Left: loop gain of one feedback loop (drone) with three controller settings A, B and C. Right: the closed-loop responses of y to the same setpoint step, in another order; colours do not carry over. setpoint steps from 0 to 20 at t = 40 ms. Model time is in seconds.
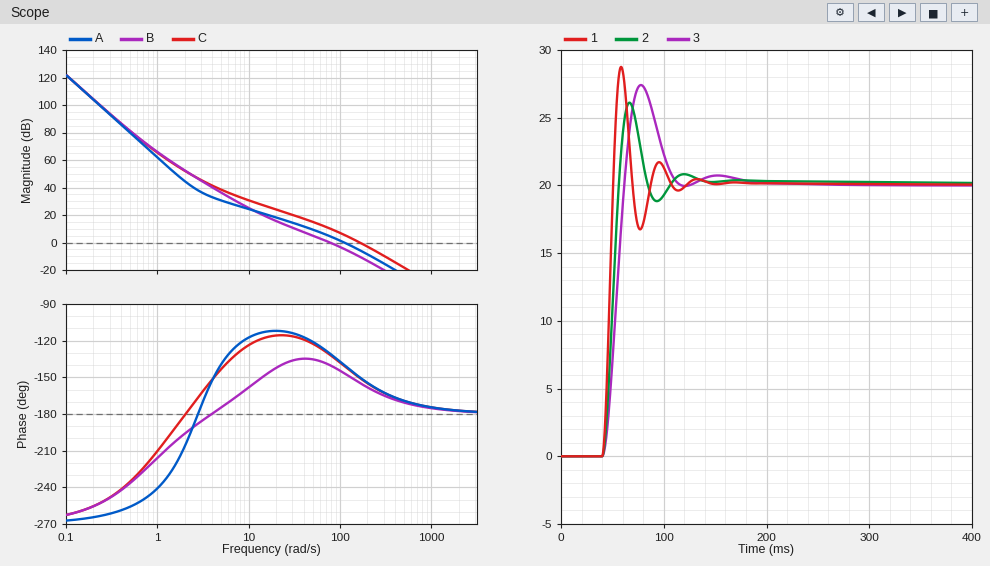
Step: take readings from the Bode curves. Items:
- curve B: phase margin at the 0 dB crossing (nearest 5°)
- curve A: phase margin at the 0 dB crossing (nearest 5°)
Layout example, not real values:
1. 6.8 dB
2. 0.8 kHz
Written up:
1. 40°
2. 40°
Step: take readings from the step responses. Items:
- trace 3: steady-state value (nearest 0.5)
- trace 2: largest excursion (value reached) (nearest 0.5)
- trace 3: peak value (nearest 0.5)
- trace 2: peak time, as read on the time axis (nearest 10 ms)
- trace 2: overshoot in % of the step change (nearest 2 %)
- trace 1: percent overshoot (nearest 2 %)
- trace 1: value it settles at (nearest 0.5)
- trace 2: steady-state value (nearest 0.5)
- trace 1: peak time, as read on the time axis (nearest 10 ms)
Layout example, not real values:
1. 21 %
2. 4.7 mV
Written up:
1. 20.0
2. 26.0
3. 27.5
4. 70 ms
5. 30 %
6. 44 %
7. 20.0
8. 20.0
9. 60 ms
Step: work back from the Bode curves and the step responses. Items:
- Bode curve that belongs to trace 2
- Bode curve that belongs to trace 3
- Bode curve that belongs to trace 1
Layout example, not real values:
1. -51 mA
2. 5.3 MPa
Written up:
1. A
2. B
3. C
